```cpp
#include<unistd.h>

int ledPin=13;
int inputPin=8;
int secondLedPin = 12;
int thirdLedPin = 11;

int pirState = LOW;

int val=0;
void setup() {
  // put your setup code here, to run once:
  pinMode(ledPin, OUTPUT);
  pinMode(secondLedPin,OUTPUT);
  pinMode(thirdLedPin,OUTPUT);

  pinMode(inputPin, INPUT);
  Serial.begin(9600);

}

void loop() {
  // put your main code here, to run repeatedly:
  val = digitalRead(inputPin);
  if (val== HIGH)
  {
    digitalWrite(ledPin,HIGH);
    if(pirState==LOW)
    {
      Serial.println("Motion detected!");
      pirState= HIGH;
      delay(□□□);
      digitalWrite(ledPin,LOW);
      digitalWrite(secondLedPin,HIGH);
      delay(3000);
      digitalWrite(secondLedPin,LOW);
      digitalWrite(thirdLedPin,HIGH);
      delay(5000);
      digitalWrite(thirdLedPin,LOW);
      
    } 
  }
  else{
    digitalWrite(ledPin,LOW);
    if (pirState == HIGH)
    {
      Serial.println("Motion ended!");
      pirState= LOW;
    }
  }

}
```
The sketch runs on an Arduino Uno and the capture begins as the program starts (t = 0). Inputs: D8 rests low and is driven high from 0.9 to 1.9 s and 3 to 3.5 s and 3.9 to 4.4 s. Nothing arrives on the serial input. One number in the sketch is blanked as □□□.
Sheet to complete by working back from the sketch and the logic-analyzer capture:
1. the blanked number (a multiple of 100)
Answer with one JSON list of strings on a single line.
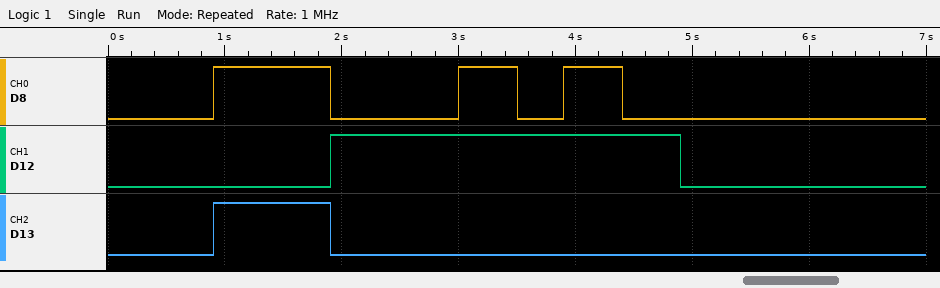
["1000"]
